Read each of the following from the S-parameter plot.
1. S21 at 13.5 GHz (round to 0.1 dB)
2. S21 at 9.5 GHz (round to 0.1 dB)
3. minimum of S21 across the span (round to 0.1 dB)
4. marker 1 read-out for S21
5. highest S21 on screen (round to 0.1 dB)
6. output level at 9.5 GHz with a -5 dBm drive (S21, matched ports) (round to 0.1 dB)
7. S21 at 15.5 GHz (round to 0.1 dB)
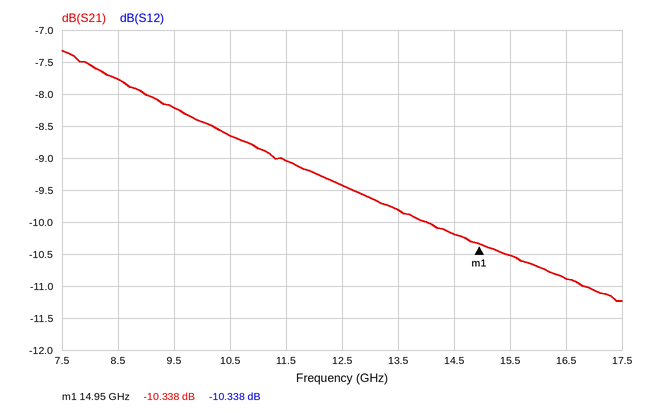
-9.8 dB
-8.2 dB
-11.2 dB
-10.338 dB
-7.3 dB
-13.2 dBm
-10.5 dB
